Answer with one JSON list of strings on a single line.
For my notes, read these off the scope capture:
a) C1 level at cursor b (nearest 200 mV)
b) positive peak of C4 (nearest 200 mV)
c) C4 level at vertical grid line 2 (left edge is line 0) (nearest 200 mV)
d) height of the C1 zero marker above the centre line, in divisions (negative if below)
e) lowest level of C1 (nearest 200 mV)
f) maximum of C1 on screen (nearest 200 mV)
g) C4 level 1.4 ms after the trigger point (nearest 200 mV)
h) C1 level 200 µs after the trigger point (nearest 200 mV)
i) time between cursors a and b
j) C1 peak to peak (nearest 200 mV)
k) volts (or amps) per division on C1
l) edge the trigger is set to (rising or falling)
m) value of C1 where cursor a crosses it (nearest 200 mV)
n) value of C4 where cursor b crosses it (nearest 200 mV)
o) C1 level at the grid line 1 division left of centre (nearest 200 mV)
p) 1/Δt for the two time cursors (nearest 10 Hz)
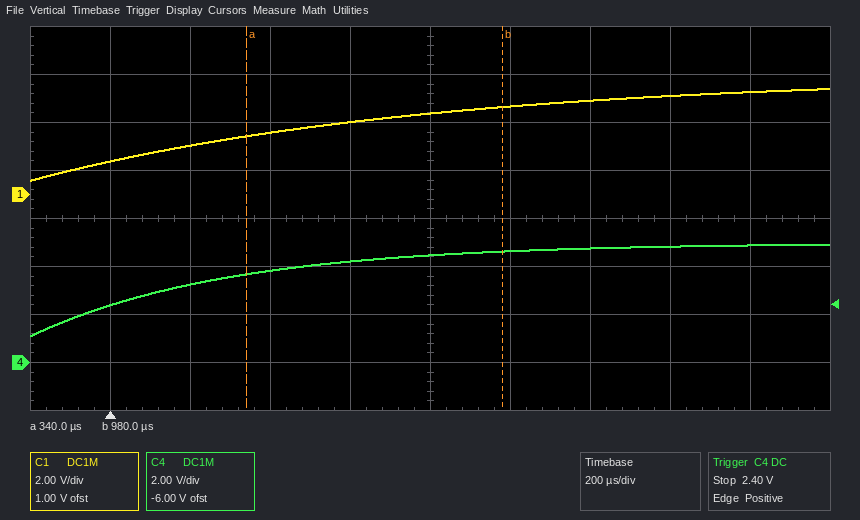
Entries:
["3.6 V", "5.0 V", "3.2 V", "+0.5 div", "600 mV", "4.4 V", "4.8 V", "2.0 V", "640 µs", "3.8 V", "2 V", "rising", "2.4 V", "4.6 V", "3.0 V", "1.56 kHz"]
